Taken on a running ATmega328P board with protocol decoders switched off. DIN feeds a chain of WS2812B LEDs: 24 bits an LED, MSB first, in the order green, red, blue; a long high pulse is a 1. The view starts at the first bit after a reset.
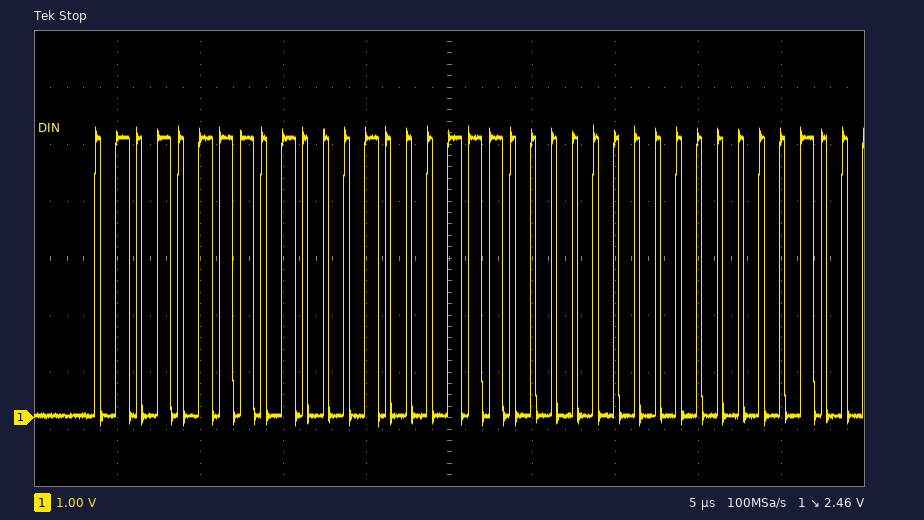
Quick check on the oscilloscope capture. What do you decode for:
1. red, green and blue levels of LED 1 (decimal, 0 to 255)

68, 87, 112
